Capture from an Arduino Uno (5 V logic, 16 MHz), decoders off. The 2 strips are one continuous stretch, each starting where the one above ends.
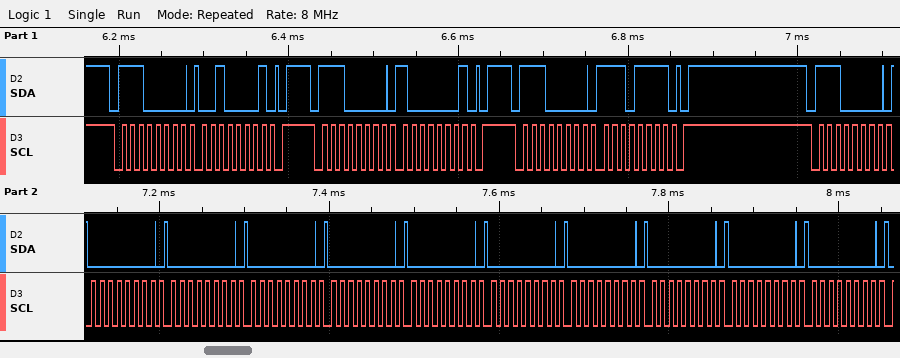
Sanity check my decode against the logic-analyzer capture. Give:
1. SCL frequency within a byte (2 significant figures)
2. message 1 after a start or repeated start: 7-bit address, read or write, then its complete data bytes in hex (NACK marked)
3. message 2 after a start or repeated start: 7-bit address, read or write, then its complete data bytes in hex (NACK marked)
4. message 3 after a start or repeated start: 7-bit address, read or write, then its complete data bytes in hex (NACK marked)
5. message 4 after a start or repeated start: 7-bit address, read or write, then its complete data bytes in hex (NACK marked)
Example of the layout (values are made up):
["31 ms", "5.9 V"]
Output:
["100 kHz", "0x70 write: 21", "0x70 write: 81", "0x70 write: EF", "0x70 write: 00 00 00 00 00 00 00 00 00 00"]
